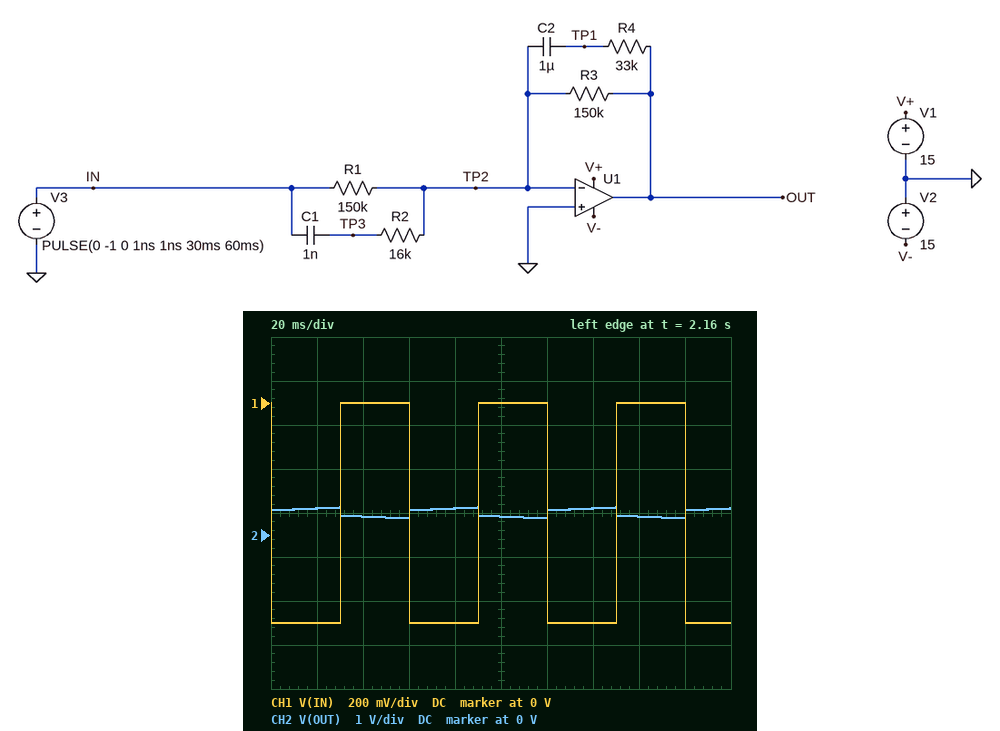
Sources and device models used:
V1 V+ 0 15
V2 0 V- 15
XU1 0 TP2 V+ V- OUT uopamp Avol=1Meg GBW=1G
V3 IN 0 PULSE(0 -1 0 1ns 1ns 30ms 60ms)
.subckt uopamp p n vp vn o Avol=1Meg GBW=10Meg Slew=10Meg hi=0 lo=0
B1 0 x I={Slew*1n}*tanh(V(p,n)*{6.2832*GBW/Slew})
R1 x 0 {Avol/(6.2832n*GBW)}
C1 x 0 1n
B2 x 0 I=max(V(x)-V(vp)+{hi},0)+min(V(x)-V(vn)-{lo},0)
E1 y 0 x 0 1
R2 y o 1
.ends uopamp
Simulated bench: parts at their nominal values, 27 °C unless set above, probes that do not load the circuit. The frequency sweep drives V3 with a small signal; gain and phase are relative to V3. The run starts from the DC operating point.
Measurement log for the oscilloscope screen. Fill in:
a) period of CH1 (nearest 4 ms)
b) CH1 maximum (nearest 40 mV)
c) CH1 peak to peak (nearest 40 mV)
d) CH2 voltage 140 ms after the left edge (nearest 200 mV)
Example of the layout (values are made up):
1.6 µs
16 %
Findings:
60 ms
0 V
1.00 V
600 mV
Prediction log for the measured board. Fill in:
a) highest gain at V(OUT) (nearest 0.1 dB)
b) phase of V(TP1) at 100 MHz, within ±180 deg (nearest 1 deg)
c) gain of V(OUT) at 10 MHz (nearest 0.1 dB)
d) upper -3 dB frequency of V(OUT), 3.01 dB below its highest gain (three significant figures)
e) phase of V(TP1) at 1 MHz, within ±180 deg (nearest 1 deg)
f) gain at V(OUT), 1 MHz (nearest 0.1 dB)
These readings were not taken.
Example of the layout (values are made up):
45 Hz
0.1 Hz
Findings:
5.4 dB
74 deg
5.4 dB
348 MHz
90 deg
5.4 dB
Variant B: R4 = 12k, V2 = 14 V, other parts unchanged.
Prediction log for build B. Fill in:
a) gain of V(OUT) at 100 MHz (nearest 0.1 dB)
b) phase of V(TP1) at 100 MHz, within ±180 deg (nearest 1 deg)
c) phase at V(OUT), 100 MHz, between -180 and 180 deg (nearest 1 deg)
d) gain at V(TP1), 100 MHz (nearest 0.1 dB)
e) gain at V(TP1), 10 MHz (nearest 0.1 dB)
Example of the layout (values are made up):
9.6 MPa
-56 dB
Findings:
-2.4 dB
80 deg
170 deg
-22.4 dB
-42.3 dB
